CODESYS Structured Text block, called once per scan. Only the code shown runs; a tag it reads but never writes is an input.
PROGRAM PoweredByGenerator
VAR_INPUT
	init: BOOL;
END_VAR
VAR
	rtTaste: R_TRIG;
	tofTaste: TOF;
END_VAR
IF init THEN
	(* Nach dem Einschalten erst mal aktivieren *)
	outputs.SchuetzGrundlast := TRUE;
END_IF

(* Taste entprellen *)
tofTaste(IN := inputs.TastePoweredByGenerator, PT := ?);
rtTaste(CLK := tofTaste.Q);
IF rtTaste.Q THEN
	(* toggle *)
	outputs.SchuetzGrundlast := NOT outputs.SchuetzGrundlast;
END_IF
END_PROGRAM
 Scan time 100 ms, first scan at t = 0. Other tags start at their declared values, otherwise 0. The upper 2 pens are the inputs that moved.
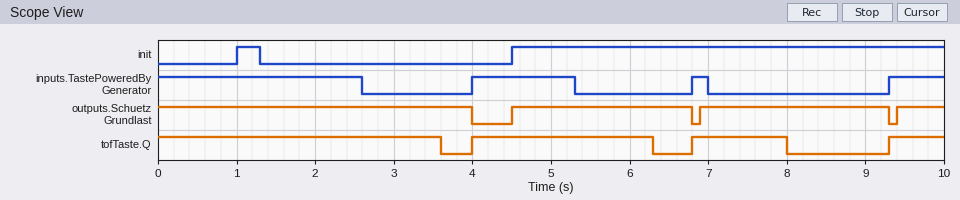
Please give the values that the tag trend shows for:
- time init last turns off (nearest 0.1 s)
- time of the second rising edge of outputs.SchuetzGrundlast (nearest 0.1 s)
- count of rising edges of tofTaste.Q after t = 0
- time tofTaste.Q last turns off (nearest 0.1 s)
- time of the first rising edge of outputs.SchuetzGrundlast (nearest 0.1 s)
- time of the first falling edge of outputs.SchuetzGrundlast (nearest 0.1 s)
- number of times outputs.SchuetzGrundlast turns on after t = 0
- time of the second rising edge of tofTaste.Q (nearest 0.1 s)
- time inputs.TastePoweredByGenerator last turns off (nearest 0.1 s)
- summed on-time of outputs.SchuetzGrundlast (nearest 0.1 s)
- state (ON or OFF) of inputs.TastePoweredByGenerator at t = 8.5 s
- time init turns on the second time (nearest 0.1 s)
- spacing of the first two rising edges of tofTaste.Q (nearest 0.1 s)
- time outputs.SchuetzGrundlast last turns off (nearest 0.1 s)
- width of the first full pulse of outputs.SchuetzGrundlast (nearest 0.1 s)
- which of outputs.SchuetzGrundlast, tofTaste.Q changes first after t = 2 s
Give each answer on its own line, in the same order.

1.3 s
6.9 s
3
8.0 s
4.5 s
4.0 s
3
6.8 s
7.0 s
9.3 s
OFF
4.5 s
2.8 s
9.3 s
2.3 s
tofTaste.Q
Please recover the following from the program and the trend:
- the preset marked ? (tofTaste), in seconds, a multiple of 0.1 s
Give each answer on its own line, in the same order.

1.0 s
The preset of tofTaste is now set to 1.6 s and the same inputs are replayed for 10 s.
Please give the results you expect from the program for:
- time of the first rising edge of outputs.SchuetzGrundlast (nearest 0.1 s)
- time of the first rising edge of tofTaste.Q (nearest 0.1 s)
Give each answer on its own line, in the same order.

9.4 s
9.3 s
